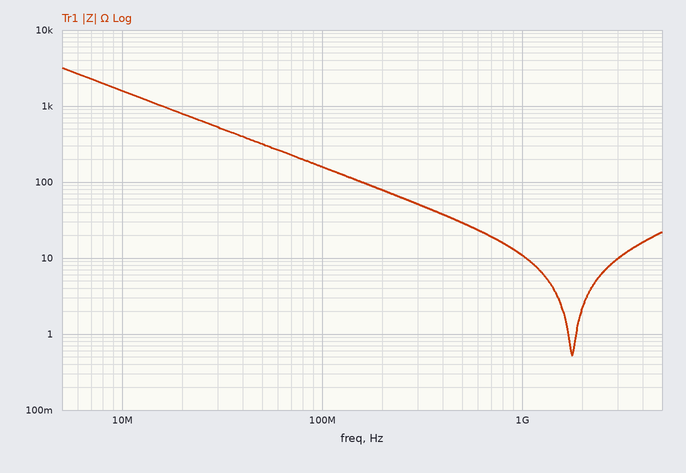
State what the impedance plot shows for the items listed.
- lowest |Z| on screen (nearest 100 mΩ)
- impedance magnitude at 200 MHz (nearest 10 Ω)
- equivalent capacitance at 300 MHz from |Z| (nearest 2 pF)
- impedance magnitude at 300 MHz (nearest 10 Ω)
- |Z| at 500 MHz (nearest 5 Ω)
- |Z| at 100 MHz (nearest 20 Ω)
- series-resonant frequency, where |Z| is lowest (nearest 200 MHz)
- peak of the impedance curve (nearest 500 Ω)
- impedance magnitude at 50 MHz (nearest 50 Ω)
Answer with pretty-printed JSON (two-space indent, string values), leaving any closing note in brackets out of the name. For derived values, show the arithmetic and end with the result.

{
  "lowest |Z| on screen": "500 mΩ",
  "impedance magnitude at 200 MHz": "80 Ω",
  "equivalent capacitance at 300 MHz from |Z|": "C = 1/(2π × 300 MHz × 50 Ω) ≈ 10.6 pF, so 10 pF to the nearest 2 pF",
  "impedance magnitude at 300 MHz": "50 Ω",
  "|Z| at 500 MHz": "30 Ω",
  "|Z| at 100 MHz": "160 Ω",
  "series-resonant frequency, where |Z| is lowest": "1.8 GHz",
  "peak of the impedance curve": "3.0 kΩ",
  "impedance magnitude at 50 MHz": "300 Ω"
}
